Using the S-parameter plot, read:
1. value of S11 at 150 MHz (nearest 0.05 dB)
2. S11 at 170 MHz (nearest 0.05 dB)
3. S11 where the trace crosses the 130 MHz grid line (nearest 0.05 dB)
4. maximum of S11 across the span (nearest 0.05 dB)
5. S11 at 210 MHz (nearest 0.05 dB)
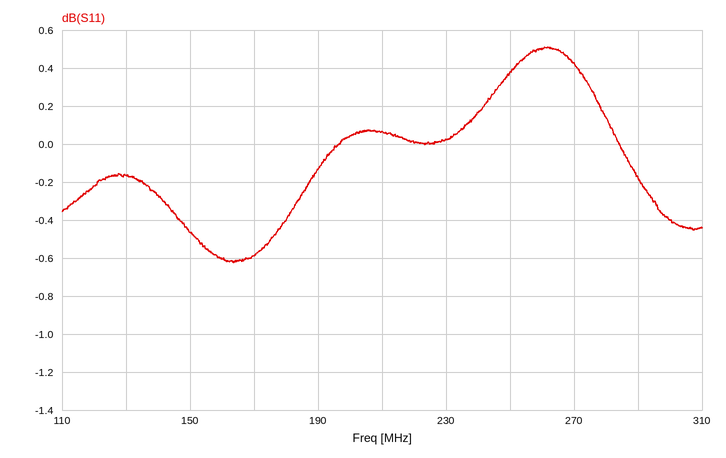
-0.45 dB
-0.60 dB
-0.15 dB
0.50 dB
0.05 dB
